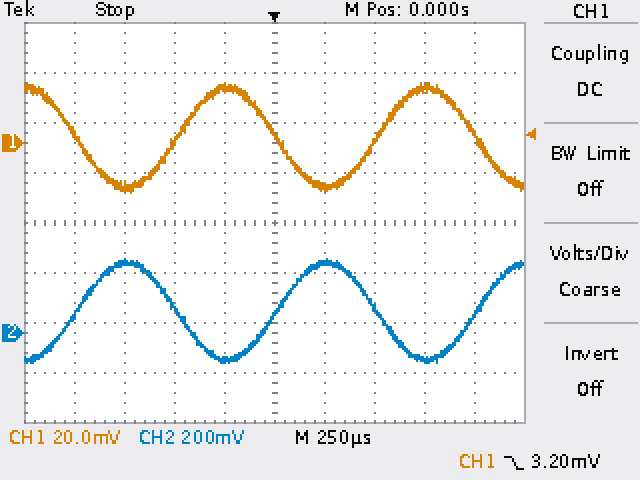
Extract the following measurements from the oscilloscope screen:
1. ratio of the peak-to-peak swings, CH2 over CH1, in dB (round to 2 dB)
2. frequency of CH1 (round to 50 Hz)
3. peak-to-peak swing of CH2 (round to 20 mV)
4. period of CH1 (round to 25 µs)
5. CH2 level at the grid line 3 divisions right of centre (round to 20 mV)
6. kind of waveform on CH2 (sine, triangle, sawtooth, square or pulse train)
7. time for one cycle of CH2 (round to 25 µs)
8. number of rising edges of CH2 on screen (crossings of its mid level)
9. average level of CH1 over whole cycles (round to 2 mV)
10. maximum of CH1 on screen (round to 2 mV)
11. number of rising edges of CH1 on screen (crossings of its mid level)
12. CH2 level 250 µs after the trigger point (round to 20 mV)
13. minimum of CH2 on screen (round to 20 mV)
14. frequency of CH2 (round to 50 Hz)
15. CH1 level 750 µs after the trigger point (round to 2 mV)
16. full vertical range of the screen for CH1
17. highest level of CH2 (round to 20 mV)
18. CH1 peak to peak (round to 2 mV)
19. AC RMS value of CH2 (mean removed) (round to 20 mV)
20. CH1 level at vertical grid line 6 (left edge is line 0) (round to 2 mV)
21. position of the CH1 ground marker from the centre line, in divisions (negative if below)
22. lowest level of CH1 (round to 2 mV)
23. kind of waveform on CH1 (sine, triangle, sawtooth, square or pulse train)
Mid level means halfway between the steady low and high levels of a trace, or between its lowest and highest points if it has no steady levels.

20 dB
1.00 kHz
420 mV
1.000 ms
-100 mV
sine
1.000 ms
3
2 mV
24 mV
2
280 mV
-120 mV
1.00 kHz
22 mV
160 mV
300 mV
44 mV
140 mV
-18 mV
+1.6 div
-20 mV
sine
